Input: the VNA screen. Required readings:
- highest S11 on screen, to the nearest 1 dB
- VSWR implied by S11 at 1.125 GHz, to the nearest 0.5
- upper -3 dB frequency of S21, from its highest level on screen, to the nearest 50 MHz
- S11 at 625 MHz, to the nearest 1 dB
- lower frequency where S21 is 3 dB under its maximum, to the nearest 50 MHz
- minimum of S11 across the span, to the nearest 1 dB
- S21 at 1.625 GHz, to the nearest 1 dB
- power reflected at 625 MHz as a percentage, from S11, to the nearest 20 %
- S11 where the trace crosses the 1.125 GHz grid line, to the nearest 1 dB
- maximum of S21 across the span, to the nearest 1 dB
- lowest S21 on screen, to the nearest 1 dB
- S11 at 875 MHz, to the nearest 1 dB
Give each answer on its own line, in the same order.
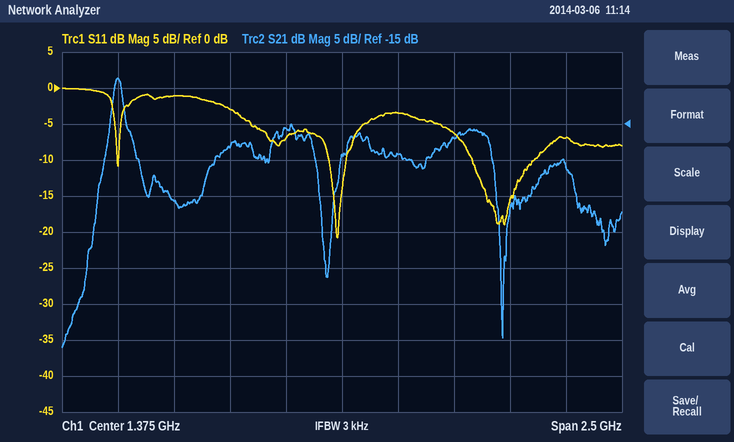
0 dB
2.5
400 MHz
-1 dB
350 MHz
-21 dB
-19 dB
80 %
-7 dB
-9 dB
-46 dB
-3 dB
